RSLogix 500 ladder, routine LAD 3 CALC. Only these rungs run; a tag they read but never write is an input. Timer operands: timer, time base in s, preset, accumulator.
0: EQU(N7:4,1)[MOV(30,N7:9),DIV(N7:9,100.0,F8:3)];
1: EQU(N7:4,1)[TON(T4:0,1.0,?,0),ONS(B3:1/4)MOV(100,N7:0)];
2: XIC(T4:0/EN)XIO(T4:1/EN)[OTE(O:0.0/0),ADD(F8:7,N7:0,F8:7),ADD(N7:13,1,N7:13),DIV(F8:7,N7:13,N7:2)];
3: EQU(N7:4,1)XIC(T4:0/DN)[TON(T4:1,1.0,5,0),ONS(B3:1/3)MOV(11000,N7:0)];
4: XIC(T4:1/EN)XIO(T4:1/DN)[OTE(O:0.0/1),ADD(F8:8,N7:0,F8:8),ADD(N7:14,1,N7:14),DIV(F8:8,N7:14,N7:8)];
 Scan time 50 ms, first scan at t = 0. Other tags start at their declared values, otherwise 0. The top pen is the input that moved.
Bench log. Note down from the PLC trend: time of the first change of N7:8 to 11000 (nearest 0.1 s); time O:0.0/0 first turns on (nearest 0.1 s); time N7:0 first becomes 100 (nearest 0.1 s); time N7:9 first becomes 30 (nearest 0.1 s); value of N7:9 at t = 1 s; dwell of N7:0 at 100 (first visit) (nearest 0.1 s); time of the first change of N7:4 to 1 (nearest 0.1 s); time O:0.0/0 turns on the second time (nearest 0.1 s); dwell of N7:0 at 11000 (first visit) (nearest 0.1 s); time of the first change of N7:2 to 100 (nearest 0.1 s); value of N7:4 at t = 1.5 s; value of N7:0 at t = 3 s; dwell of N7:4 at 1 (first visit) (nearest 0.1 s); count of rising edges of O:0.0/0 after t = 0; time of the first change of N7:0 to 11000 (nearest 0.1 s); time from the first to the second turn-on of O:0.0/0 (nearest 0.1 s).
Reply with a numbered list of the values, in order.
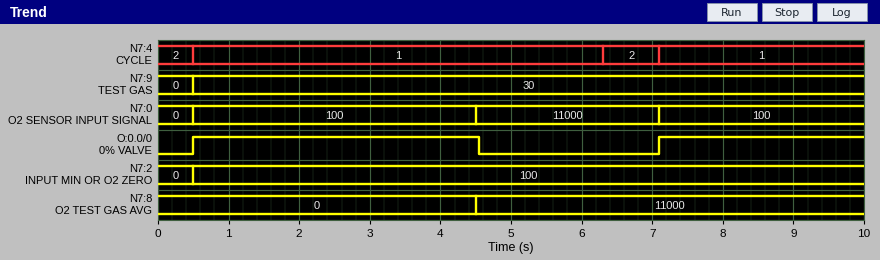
1. 4.5 s
2. 0.5 s
3. 0.5 s
4. 0.5 s
5. 30
6. 4.0 s
7. 0.5 s
8. 7.1 s
9. 2.6 s
10. 0.5 s
11. 1
12. 100
13. 5.8 s
14. 2
15. 4.5 s
16. 6.6 s
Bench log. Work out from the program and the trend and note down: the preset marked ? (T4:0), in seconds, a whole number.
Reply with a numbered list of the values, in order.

1. 4 s
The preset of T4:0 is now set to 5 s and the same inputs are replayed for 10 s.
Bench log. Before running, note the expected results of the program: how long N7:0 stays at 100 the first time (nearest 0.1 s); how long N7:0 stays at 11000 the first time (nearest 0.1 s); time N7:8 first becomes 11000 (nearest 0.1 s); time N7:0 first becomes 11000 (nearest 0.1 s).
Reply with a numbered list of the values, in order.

1. 5.0 s
2. 1.6 s
3. 5.5 s
4. 5.5 s
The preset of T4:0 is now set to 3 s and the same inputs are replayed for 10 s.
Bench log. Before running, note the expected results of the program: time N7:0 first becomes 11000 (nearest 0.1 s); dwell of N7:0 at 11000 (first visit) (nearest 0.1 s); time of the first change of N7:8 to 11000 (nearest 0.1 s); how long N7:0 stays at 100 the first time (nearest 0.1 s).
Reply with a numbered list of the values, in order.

1. 3.5 s
2. 3.6 s
3. 3.5 s
4. 3.0 s
